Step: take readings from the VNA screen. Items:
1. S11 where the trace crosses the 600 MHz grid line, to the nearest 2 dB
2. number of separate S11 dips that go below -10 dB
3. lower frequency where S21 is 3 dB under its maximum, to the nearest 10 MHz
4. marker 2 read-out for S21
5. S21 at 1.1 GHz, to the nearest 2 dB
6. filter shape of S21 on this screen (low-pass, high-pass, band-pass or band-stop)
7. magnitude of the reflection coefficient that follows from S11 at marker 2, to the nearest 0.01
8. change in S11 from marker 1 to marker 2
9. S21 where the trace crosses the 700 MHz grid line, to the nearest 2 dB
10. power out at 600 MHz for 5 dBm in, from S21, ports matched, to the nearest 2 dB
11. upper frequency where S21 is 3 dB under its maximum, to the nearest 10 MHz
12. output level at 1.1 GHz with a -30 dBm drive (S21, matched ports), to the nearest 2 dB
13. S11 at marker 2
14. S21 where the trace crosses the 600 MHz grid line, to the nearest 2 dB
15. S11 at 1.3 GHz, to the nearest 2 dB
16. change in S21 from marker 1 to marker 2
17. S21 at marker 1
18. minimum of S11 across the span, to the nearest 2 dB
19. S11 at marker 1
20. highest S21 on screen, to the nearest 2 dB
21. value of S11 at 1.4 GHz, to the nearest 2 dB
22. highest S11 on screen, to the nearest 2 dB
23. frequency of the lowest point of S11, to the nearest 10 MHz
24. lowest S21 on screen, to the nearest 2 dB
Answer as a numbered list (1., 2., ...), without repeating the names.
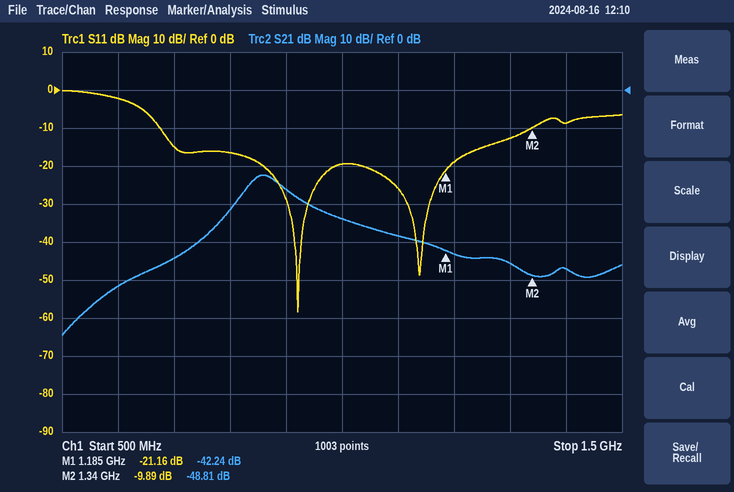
1. -2 dB
2. 2
3. 830 MHz
4. -48.81 dB
5. -38 dB
6. band-pass
7. 0.32
8. 11.27 dB
9. -44 dB
10. -46 dBm
11. 890 MHz
12. -68 dBm
13. -9.89 dB
14. -52 dB
15. -12 dB
16. -6.57 dB
17. -42.24 dB
18. -58 dB
19. -21.16 dB
20. -22 dB
21. -8 dB
22. 0 dB
23. 920 MHz
24. -64 dB
